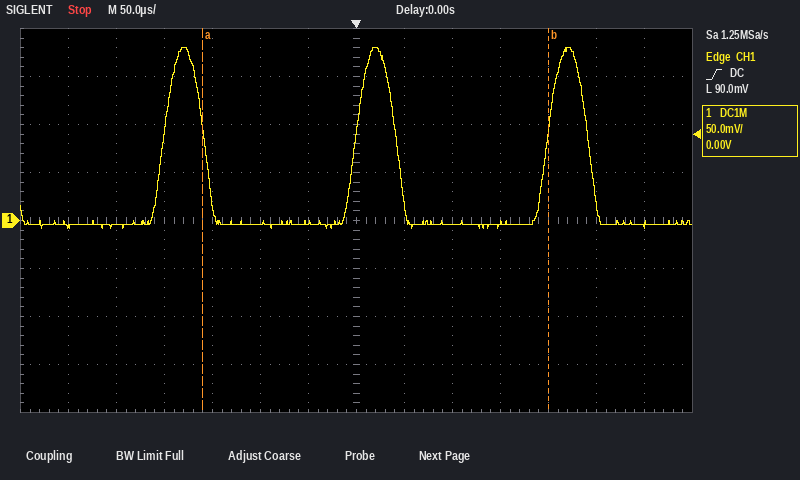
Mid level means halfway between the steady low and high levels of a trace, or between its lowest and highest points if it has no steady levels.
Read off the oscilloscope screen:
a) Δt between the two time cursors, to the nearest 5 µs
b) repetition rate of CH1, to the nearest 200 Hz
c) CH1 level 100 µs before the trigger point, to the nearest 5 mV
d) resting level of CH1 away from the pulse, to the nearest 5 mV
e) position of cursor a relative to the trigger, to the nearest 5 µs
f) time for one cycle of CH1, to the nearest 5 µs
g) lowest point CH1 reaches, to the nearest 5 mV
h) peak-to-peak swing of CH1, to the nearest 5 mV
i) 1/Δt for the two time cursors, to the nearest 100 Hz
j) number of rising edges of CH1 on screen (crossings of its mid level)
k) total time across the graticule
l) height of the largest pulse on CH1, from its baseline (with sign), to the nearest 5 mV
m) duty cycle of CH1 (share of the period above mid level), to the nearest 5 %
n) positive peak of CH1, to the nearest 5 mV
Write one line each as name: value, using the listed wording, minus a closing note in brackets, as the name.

Δt between the two time cursors, to the nearest 5 µs: 360 µs
repetition rate of CH1, to the nearest 200 Hz: 5.0 kHz
CH1 level 100 µs before the trigger point, to the nearest 5 mV: -5 mV
resting level of CH1 away from the pulse, to the nearest 5 mV: -5 mV
position of cursor a relative to the trigger, to the nearest 5 µs: -160 µs
time for one cycle of CH1, to the nearest 5 µs: 200 µs
lowest point CH1 reaches, to the nearest 5 mV: -10 mV
peak-to-peak swing of CH1, to the nearest 5 mV: 190 mV
1/Δt for the two time cursors, to the nearest 100 Hz: 2.8 kHz
number of rising edges of CH1 on screen: 3
total time across the graticule: 700 µs
height of the largest pulse on CH1, from its baseline (with sign), to the nearest 5 mV: +185 mV
duty cycle of CH1 (share of the period above mid level), to the nearest 5 %: 20 %
positive peak of CH1, to the nearest 5 mV: 180 mV
